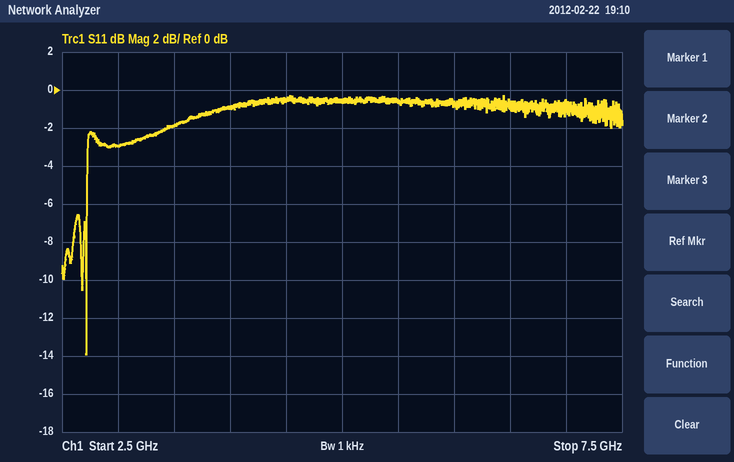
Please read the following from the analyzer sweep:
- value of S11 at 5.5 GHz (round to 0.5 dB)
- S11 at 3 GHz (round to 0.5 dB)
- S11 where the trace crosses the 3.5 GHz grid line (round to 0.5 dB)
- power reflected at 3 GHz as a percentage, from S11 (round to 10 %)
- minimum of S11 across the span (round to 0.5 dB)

-0.5 dB
-3.0 dB
-2.0 dB
50 %
-14.0 dB
